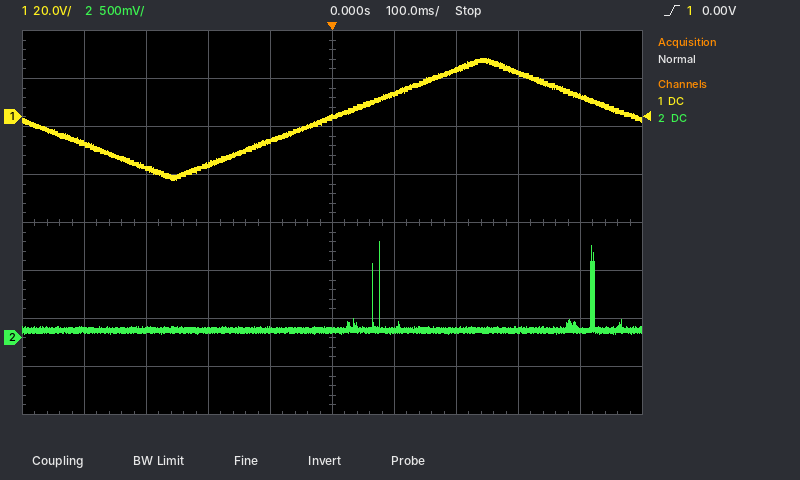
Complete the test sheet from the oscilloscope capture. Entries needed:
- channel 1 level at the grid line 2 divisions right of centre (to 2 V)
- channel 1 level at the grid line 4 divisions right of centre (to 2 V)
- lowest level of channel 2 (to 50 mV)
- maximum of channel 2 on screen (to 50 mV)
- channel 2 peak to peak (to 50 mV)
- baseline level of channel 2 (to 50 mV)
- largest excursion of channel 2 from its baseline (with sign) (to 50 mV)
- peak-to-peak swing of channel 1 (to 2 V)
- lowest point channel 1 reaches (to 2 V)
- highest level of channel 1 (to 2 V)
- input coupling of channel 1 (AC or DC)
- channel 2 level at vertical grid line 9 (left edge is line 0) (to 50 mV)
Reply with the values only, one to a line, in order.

20 V
8 V
50 mV
1.00 V
950 mV
100 mV
+900 mV
50 V
-26 V
24 V
DC
100 mV
